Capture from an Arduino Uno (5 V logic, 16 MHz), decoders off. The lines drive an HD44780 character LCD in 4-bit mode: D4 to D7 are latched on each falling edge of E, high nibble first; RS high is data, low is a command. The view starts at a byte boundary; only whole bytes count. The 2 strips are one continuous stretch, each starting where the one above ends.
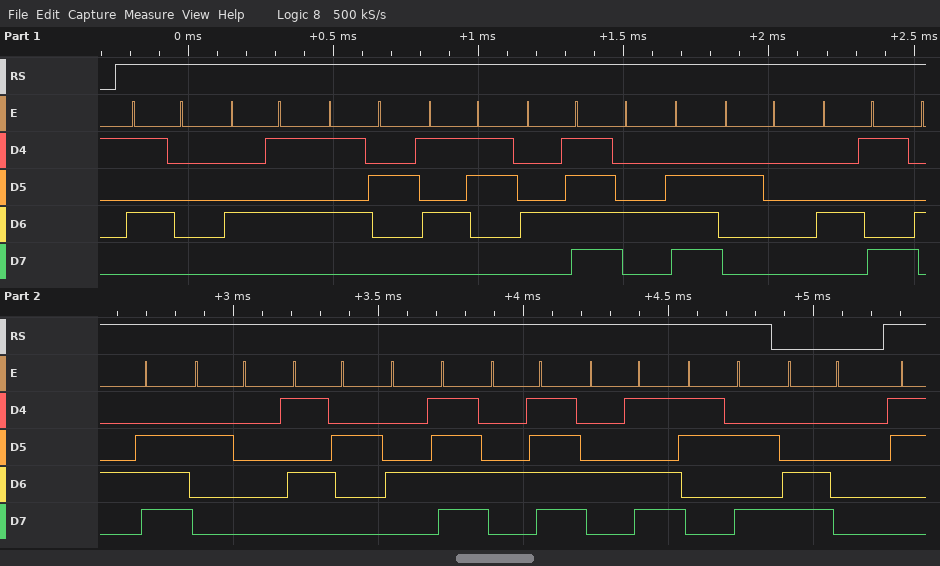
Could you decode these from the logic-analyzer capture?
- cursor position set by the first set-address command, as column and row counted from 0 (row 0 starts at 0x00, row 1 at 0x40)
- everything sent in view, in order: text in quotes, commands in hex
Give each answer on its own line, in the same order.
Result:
column 0, row 1
"PERSON IN ROOM:" 0xC0
